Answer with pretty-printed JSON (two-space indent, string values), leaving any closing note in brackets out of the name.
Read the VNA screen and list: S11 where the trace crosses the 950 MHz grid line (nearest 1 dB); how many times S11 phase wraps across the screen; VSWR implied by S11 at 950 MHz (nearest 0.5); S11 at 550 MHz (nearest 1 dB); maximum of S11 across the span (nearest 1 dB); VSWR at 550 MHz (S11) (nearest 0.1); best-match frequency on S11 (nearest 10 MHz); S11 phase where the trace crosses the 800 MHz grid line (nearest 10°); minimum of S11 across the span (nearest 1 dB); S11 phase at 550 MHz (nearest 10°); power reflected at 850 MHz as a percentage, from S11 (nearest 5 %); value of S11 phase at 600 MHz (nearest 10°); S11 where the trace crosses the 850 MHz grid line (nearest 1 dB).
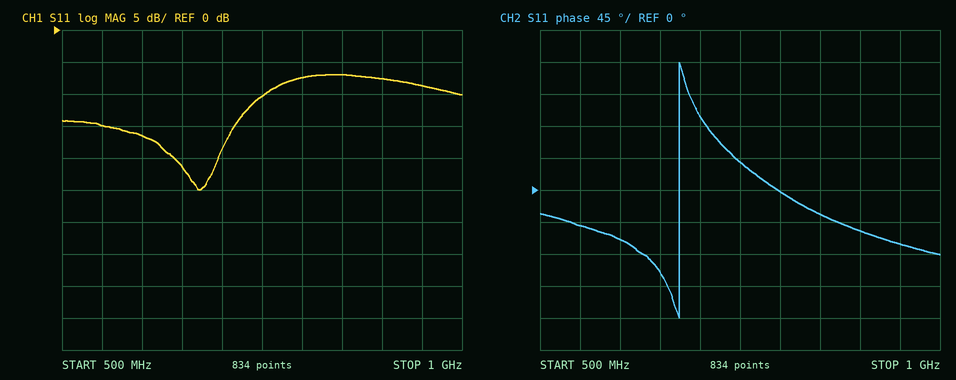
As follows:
{
  "S11 where the trace crosses the 950 MHz grid line": "-9 dB",
  "how many times S11 phase wraps across the screen": "1",
  "VSWR implied by S11 at 950 MHz": "2.0",
  "S11 at 550 MHz": "-15 dB",
  "maximum of S11 across the span": "-7 dB",
  "VSWR at 550 MHz (S11)": "1.4",
  "best-match frequency on S11": "670 MHz",
  "S11 phase where the trace crosses the 800 MHz grid line": "0°",
  "minimum of S11 across the span": "-25 dB",
  "S11 phase at 550 MHz": "-50°",
  "power reflected at 850 MHz as a percentage, from S11": "20 %",
  "value of S11 phase at 600 MHz": "-70°",
  "S11 where the trace crosses the 850 MHz grid line": "-7 dB"
}
